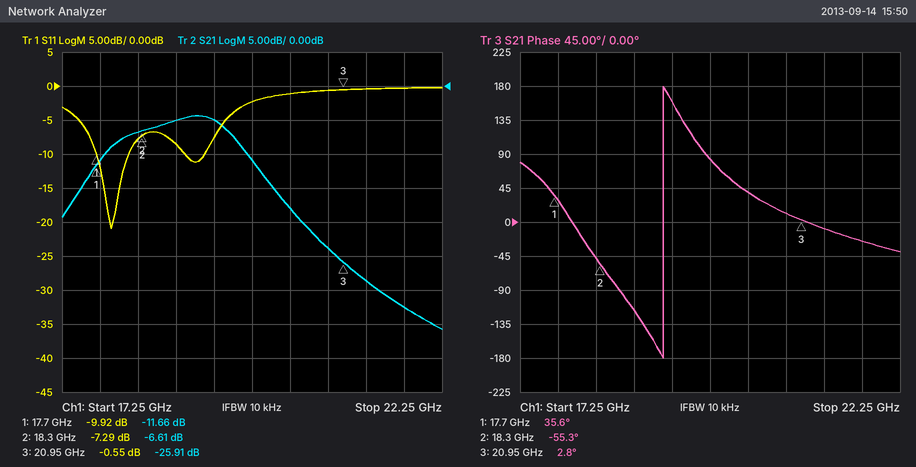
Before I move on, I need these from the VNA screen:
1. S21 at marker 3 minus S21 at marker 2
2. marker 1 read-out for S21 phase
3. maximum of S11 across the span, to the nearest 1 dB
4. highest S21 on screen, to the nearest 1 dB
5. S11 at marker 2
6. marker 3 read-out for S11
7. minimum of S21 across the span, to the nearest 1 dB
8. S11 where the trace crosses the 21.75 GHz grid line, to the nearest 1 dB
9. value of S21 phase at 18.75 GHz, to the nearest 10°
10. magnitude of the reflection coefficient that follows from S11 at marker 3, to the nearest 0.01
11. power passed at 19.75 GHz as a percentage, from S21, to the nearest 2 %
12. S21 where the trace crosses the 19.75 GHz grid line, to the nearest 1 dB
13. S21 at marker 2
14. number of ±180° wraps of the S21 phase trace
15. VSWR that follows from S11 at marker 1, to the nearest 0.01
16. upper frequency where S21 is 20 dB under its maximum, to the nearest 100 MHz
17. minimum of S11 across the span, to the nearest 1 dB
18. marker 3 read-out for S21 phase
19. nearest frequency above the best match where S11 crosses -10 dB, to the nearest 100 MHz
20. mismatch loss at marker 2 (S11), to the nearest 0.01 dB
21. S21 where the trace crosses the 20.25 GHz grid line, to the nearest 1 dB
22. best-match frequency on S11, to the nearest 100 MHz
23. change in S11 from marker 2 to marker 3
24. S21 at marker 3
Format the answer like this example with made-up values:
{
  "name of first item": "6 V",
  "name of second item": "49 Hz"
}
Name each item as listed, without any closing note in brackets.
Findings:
{
  "S21 at marker 3 minus S21 at marker 2": "-19.30 dB",
  "marker 1 read-out for S21 phase": "35.6°",
  "maximum of S11 across the span, to the nearest 1 dB": "0 dB",
  "highest S21 on screen, to the nearest 1 dB": "-4 dB",
  "S11 at marker 2": "-7.29 dB",
  "marker 3 read-out for S11": "-0.55 dB",
  "minimum of S21 across the span, to the nearest 1 dB": "-36 dB",
  "S11 where the trace crosses the 21.75 GHz grid line, to the nearest 1 dB": "0 dB",
  "value of S21 phase at 18.75 GHz, to the nearest 10°": "-120°",
  "magnitude of the reflection coefficient that follows from S11 at marker 3, to the nearest 0.01": "0.94",
  "power passed at 19.75 GHz as a percentage, from S21, to the nearest 2 %": "8 %",
  "S21 where the trace crosses the 19.75 GHz grid line, to the nearest 1 dB": "-11 dB",
  "S21 at marker 2": "-6.61 dB",
  "number of ±180° wraps of the S21 phase trace": "1",
  "VSWR that follows from S11 at marker 1, to the nearest 0.01": "1.94",
  "upper frequency where S21 is 20 dB under its maximum, to the nearest 100 MHz": "20.8 GHz",
  "minimum of S11 across the span, to the nearest 1 dB": "-21 dB",
  "marker 3 read-out for S21 phase": "2.8°",
  "nearest frequency above the best match where S11 crosses -10 dB, to the nearest 100 MHz": "18.1 GHz",
  "mismatch loss at marker 2 (S11), to the nearest 0.01 dB": "0.90 dB",
  "S21 where the trace crosses the 20.25 GHz grid line, to the nearest 1 dB": "-18 dB",
  "best-match frequency on S11, to the nearest 100 MHz": "17.9 GHz",
  "change in S11 from marker 2 to marker 3": "6.74 dB",
  "S21 at marker 3": "-25.91 dB"
}
